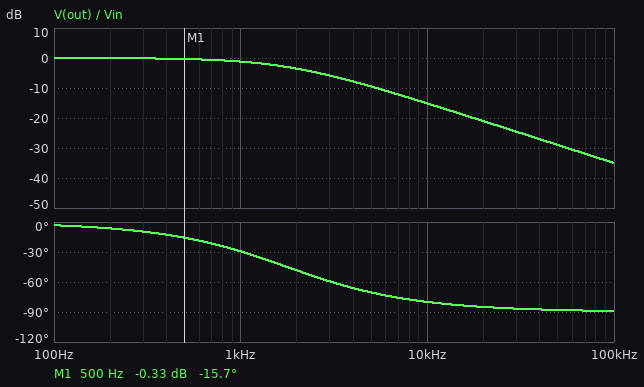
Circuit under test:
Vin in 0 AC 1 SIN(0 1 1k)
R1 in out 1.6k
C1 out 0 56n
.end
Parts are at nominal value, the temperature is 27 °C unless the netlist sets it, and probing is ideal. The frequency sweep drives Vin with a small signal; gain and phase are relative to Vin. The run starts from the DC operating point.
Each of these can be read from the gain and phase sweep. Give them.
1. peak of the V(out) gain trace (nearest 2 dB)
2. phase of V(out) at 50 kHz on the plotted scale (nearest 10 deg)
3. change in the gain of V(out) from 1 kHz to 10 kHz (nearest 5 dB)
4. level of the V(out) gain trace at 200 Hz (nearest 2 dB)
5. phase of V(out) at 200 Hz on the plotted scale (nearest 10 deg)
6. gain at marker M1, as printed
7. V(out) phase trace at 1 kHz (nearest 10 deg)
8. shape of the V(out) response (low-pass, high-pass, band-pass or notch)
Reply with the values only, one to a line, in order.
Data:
0 dB
-90 deg
-15 dB
0 dB
-10 deg
-0.33 dB
-30 deg
low-pass
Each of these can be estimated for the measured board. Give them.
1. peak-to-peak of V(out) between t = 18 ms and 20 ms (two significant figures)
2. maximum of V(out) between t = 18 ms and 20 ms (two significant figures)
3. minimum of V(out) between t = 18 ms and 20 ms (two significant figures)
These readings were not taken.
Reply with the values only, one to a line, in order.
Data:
1.7 V
870 mV
-870 mV
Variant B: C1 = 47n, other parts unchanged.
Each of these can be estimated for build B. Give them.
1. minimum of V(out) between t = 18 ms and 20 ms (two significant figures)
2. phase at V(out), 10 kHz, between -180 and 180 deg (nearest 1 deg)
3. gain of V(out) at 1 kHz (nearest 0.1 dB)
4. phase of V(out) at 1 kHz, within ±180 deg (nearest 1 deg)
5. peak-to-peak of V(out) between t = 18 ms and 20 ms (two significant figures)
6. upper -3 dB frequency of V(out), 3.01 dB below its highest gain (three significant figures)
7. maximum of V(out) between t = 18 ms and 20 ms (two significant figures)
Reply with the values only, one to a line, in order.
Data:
-900 mV
-78 deg
-0.9 dB
-25 deg
1.8 V
2.12 kHz
900 mV
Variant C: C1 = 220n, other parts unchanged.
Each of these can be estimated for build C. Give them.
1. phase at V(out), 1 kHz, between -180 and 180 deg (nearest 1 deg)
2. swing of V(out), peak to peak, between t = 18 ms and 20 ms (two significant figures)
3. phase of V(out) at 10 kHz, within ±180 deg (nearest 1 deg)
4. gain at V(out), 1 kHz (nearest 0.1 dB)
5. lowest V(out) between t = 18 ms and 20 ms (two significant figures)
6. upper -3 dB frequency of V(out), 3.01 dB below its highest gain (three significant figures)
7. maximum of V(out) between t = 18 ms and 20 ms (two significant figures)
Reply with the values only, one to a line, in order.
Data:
-66 deg
820 mV
-87 deg
-7.7 dB
-410 mV
452 Hz
410 mV
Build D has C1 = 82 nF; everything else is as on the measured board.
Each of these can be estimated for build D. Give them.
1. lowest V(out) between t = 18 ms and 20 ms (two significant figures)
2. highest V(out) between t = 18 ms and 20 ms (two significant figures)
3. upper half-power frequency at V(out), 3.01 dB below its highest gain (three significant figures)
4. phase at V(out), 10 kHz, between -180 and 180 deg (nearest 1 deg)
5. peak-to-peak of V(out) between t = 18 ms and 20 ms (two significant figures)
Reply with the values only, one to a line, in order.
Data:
-770 mV
770 mV
1.21 kHz
-83 deg
1.5 V
